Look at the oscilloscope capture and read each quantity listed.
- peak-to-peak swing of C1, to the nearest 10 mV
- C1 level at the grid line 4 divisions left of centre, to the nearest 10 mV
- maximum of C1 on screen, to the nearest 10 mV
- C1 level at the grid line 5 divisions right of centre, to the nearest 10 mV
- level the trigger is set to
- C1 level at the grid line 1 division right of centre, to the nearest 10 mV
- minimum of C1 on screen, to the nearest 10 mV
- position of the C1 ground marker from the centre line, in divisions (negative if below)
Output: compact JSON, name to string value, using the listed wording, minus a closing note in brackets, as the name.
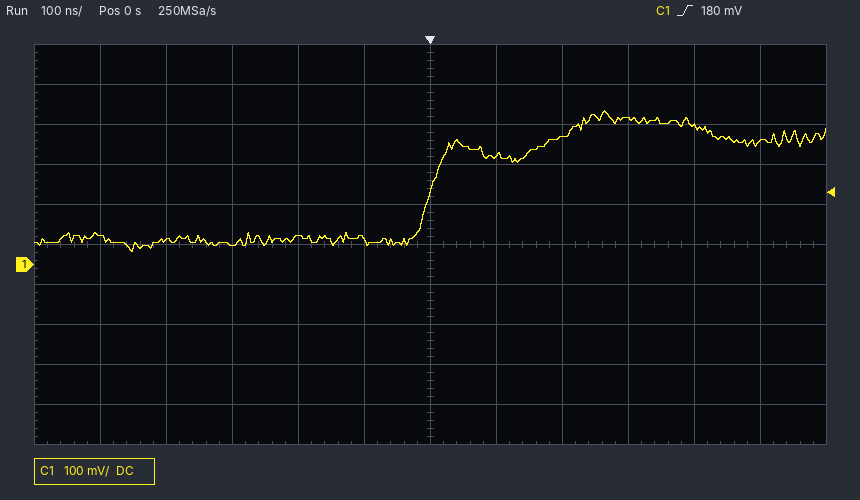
{"peak-to-peak swing of C1, to the nearest 10 mV": "350 mV", "C1 level at the grid line 4 divisions left of centre, to the nearest 10 mV": "60 mV", "maximum of C1 on screen, to the nearest 10 mV": "380 mV", "C1 level at the grid line 5 divisions right of centre, to the nearest 10 mV": "310 mV", "level the trigger is set to": "180 mV", "C1 level at the grid line 1 division right of centre, to the nearest 10 mV": "270 mV", "minimum of C1 on screen, to the nearest 10 mV": "30 mV", "position of the C1 ground marker from the centre line, in divisions": "-0.5 div"}
